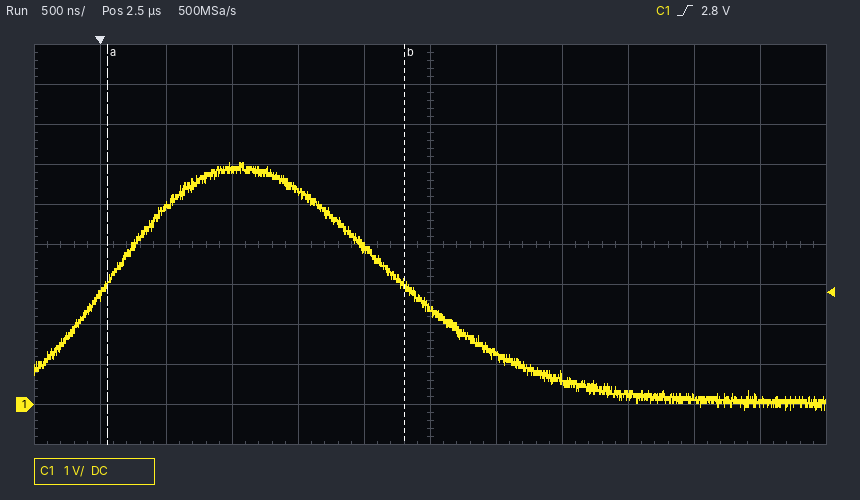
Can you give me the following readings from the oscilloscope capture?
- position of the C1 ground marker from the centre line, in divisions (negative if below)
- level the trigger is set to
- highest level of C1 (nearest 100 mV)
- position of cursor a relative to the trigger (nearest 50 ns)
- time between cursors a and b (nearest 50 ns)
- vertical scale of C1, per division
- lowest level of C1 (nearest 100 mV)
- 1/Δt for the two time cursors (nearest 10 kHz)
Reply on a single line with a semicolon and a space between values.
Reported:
-4.0 div; 2.8 V; 6.0 V; +50 ns; 2.25 µs; 1 V; -100 mV; 440 kHz
